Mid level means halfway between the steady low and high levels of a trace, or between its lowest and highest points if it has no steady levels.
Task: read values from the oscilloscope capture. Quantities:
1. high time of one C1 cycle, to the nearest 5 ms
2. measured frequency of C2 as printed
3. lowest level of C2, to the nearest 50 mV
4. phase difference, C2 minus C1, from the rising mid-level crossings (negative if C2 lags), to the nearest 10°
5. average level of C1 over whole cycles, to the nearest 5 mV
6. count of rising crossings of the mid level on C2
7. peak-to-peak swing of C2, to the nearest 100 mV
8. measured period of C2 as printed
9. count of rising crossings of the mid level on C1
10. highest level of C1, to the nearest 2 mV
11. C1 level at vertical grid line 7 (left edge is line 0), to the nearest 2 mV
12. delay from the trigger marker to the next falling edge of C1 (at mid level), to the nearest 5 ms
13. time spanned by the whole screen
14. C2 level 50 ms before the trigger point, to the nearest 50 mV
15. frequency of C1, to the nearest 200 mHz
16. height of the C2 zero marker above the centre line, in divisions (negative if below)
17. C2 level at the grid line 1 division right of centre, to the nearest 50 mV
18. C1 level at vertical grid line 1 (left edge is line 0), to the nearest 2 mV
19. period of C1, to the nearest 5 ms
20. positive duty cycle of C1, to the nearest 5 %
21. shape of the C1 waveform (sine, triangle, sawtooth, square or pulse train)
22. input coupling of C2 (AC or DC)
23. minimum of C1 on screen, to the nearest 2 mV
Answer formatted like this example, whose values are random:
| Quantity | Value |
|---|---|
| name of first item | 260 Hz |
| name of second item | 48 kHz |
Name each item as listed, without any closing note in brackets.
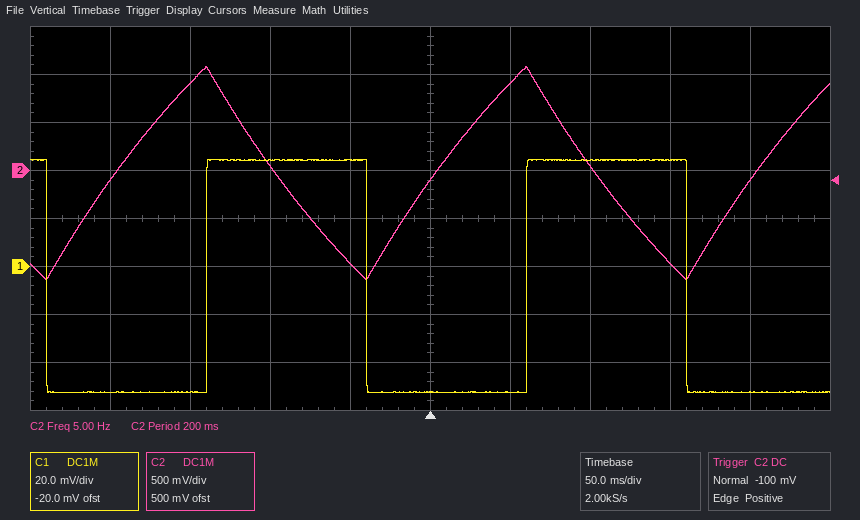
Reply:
| Quantity | Value |
|---|---|
| high time of one C1 cycle, to the nearest 5 ms | 100 ms |
| measured frequency of C2 as printed | 5.00 Hz |
| lowest level of C2, to the nearest 50 mV | -1.15 V |
| phase difference, C2 minus C1, from the rising mid-level crossings (negative if C2 lags), to the nearest 10° | +100° |
| average level of C1 over whole cycles, to the nearest 5 mV | -5 mV |
| count of rising crossings of the mid level on C2 | 3 |
| peak-to-peak swing of C2, to the nearest 100 mV | 2.20 V |
| measured period of C2 as printed | 200 ms |
| count of rising crossings of the mid level on C1 | 2 |
| highest level of C1, to the nearest 2 mV | 44 mV |
| C1 level at vertical grid line 7 (left edge is line 0), to the nearest 2 mV | 44 mV |
| delay from the trigger marker to the next falling edge of C1 (at mid level), to the nearest 5 ms | 160 ms |
| time spanned by the whole screen | 500 ms |
| C2 level 50 ms before the trigger point, to the nearest 50 mV | -950 mV |
| frequency of C1, to the nearest 200 mHz | 5.0 Hz |
| height of the C2 zero marker above the centre line, in divisions | +1.0 div |
| C2 level at the grid line 1 division right of centre, to the nearest 50 mV | 900 mV |
| C1 level at vertical grid line 1 (left edge is line 0), to the nearest 2 mV | -52 mV |
| period of C1, to the nearest 5 ms | 200 ms |
| positive duty cycle of C1, to the nearest 5 % | 50 % |
| shape of the C1 waveform | square |
| input coupling of C2 | DC |
| minimum of C1 on screen, to the nearest 2 mV | -52 mV |
